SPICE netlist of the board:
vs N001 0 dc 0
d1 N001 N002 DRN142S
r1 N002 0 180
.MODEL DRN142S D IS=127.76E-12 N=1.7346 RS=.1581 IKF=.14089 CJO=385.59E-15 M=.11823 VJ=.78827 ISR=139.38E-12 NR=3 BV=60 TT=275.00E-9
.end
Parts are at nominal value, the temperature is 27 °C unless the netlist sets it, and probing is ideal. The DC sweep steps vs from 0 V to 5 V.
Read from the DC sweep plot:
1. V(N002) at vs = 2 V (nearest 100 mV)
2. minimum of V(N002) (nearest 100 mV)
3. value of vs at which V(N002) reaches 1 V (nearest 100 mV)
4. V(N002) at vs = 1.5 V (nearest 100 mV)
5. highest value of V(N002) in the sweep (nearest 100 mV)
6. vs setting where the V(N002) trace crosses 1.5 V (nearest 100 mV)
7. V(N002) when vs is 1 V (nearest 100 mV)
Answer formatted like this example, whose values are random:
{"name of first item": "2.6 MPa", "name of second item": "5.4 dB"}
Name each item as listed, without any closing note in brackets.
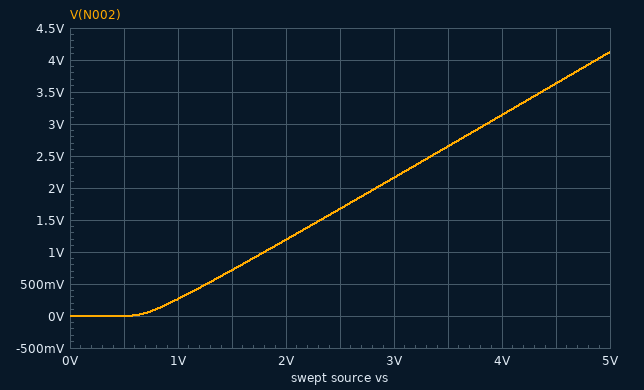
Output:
{"V(N002) at vs = 2 V": "1.2 V", "minimum of V(N002)": "0 V", "value of vs at which V(N002) reaches 1 V": "1.8 V", "V(N002) at vs = 1.5 V": "700 mV", "highest value of V(N002) in the sweep": "4.1 V", "vs setting where the V(N002) trace crosses 1.5 V": "2.3 V", "V(N002) when vs is 1 V": "300 mV"}
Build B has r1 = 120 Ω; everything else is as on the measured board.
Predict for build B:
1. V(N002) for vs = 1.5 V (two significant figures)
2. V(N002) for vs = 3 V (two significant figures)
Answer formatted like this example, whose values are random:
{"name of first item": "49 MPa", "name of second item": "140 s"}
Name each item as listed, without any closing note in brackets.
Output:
{"V(N002) for vs = 1.5 V": "700 mV", "V(N002) for vs = 3 V": "2.1 V"}
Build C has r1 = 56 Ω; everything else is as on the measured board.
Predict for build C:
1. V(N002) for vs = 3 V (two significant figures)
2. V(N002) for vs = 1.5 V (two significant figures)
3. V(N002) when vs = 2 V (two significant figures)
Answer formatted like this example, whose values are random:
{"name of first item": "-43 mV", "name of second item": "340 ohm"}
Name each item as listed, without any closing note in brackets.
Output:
{"V(N002) for vs = 3 V": "2.1 V", "V(N002) for vs = 1.5 V": "660 mV", "V(N002) when vs = 2 V": "1.1 V"}
